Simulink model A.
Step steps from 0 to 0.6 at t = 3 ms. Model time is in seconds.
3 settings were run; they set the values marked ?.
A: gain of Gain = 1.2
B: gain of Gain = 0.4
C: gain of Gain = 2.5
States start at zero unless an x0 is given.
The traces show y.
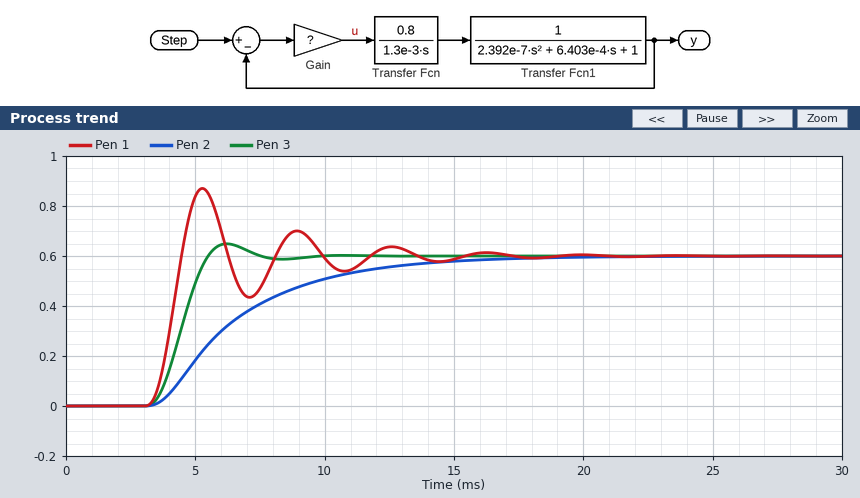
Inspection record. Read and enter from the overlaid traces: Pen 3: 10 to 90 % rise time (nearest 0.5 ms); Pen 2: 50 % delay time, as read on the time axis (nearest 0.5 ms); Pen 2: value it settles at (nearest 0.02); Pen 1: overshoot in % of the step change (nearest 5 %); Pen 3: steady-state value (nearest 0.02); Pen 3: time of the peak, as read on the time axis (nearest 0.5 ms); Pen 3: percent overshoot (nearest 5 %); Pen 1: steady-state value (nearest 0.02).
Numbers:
1.5 ms
6.0 ms
0.60
45 %
0.60
6.0 ms
10 %
0.60
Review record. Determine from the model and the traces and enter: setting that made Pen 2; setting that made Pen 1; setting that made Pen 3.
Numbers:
B
C
A
